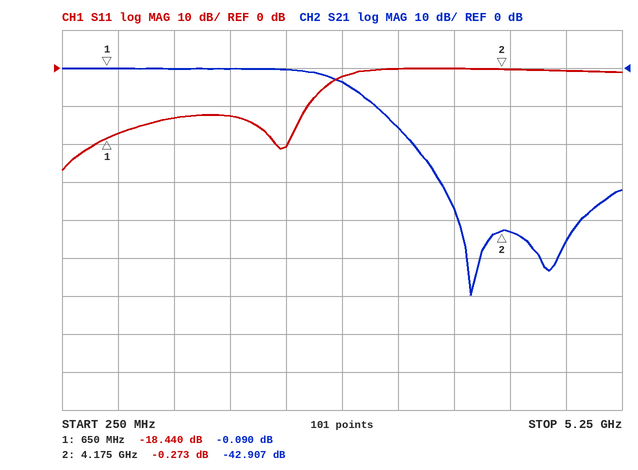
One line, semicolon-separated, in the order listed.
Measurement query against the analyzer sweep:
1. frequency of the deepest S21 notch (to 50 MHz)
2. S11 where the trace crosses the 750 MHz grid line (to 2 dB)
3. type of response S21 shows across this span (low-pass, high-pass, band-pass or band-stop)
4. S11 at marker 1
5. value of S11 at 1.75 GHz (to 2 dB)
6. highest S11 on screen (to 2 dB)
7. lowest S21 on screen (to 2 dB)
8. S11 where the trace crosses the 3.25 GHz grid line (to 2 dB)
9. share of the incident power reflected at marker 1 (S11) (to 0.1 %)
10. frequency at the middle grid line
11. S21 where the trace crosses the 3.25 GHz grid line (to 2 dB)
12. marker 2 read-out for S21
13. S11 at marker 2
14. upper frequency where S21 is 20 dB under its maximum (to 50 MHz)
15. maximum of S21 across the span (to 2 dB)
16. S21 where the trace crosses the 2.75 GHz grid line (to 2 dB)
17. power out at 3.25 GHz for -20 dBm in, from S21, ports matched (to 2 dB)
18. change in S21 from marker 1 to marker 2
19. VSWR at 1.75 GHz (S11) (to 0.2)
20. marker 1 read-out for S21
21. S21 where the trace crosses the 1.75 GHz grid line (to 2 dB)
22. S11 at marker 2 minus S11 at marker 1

3.90 GHz; -18 dB; low-pass; -18.440 dB; -12 dB; 0 dB; -60 dB; 0 dB; 1.4 %; 2.75 GHz; -16 dB; -42.907 dB; -0.273 dB; 3.40 GHz; 0 dB; -4 dB; -36 dBm; -42.817 dB; 1.6; -0.090 dB; 0 dB; 18.167 dB
